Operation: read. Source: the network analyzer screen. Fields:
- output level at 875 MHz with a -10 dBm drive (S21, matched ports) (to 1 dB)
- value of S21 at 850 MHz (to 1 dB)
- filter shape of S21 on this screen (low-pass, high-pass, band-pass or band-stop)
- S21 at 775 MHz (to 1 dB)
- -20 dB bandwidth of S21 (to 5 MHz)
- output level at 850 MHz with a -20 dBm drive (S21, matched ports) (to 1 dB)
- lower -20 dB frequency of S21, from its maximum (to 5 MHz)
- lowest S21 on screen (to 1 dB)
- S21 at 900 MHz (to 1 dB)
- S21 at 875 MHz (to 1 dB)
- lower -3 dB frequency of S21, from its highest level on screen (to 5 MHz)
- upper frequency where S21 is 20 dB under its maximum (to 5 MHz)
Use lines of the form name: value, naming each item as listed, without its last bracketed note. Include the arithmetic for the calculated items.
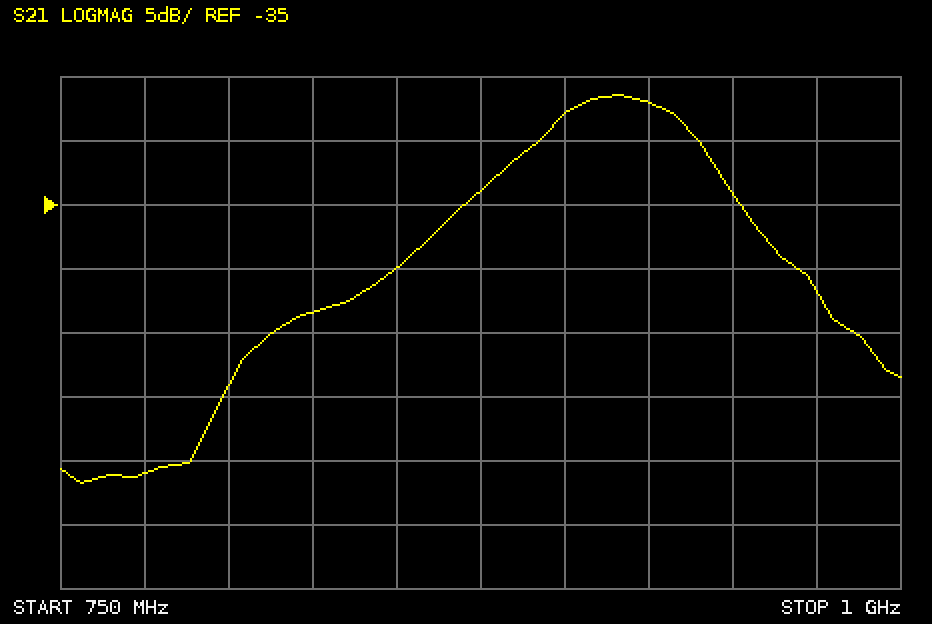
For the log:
output level at 875 MHz with a -10 dBm drive (S21, matched ports): -10 dBm + (-34 dB) = -44 dBm
value of S21 at 850 MHz: -40 dB
filter shape of S21 on this screen: band-pass
S21 at 775 MHz: -56 dB
-20 dB bandwidth of S21: 990 MHz − 805 MHz = 185 MHz
output level at 850 MHz with a -20 dBm drive (S21, matched ports): -20 dBm + (-40 dB) = -60 dBm
lower -20 dB frequency of S21, from its maximum: 805 MHz
lowest S21 on screen: -57 dB
S21 at 900 MHz: -28 dB
S21 at 875 MHz: -34 dB
lower -3 dB frequency of S21, from its highest level on screen: 895 MHz
upper frequency where S21 is 20 dB under its maximum: 990 MHz
